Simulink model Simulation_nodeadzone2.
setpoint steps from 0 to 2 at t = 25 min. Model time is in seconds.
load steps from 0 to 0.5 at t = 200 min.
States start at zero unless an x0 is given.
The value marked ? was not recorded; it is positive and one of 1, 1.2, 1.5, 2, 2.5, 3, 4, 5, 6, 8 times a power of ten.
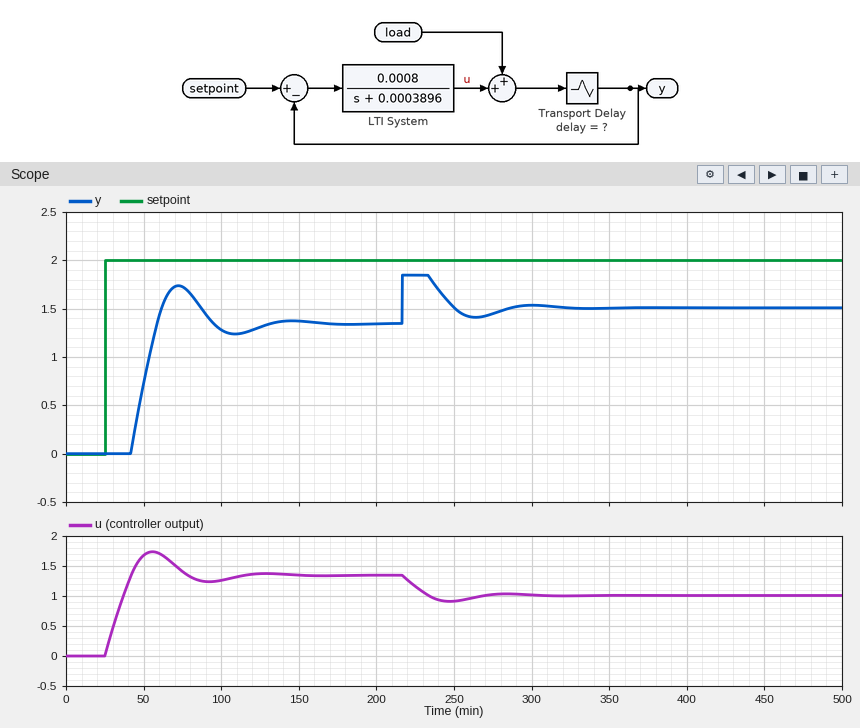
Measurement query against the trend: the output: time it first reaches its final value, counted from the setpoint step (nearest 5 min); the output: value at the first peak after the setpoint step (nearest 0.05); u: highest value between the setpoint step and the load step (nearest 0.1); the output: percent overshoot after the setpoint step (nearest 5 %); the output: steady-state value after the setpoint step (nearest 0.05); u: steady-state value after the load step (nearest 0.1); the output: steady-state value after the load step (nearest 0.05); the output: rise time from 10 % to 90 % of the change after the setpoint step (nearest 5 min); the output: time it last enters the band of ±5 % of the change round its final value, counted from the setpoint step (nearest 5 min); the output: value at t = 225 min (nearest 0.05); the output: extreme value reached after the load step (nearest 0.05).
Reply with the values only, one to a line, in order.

35 min
1.75
1.7
30 %
1.35
1.0
1.50
15 min
95 min
1.85
1.85
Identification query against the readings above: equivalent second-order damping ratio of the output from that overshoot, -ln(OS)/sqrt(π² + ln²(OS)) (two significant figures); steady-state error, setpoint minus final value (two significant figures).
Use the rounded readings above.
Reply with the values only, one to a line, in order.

0.36
0.65
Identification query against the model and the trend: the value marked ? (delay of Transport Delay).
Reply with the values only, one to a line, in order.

1000
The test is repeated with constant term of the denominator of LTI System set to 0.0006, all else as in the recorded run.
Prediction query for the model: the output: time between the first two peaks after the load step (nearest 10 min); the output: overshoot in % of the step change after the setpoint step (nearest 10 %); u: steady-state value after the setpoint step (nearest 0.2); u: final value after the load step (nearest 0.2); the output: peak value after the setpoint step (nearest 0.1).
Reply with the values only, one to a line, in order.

80 min
30 %
1.2
0.8
1.5
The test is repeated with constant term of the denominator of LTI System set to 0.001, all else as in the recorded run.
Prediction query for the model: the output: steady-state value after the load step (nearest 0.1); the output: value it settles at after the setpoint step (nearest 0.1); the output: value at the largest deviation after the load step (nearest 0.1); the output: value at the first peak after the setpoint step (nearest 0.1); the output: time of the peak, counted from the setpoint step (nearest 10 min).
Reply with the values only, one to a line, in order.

1.2
0.9
1.4
1.1
40 min
